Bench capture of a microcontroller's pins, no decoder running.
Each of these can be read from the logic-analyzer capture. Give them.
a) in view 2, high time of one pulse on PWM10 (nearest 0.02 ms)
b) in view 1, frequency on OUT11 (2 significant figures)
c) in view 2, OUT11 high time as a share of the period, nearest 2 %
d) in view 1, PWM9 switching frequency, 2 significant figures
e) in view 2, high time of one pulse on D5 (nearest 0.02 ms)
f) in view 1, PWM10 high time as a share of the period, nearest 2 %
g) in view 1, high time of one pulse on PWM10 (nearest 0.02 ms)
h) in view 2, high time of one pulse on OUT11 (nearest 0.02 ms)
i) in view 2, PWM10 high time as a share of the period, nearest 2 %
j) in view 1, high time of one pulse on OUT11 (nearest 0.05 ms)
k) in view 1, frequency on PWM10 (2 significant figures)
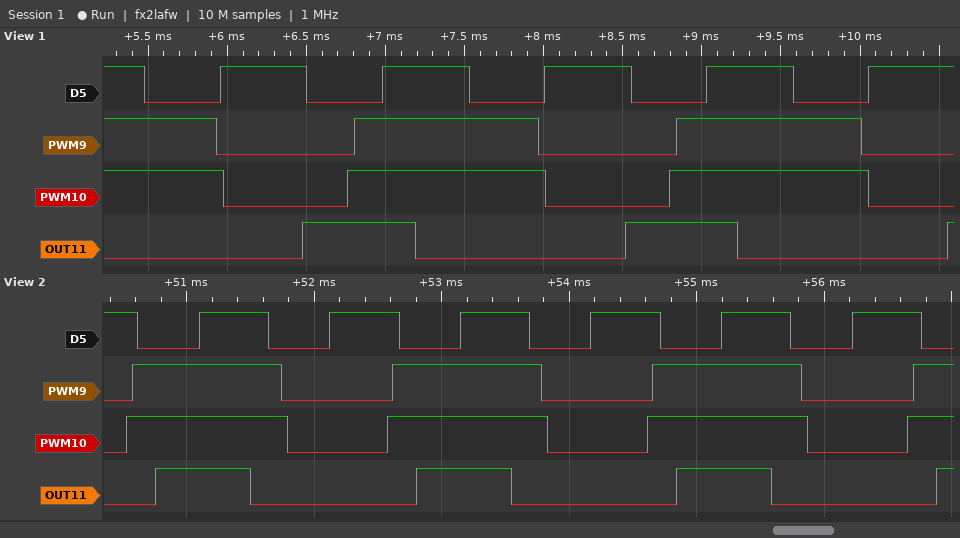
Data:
1.26 ms
490 Hz
36 %
490 Hz
0.54 ms
62 %
1.26 ms
0.74 ms
62 %
0.70 ms
490 Hz
